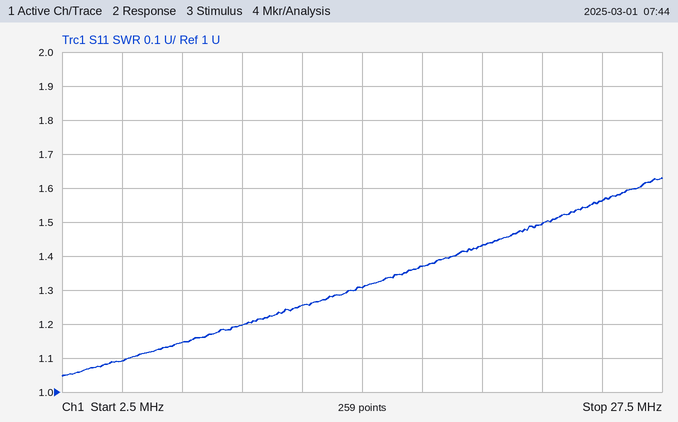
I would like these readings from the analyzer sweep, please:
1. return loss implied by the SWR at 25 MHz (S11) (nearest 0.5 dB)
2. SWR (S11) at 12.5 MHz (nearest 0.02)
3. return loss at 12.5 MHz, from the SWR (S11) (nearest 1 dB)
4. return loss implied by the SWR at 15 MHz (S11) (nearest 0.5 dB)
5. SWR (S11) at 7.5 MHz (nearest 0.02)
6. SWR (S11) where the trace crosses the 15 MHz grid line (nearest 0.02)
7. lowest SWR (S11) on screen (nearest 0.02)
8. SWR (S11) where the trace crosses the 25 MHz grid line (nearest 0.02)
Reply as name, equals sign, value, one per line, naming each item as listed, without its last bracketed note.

return loss implied by the SWR at 25 MHz (S11) = 13.0 dB
SWR (S11) at 12.5 MHz = 1.26
return loss at 12.5 MHz, from the SWR (S11) = 19 dB
return loss implied by the SWR at 15 MHz (S11) = 17.5 dB
SWR (S11) at 7.5 MHz = 1.14
SWR (S11) where the trace crosses the 15 MHz grid line = 1.30
lowest SWR (S11) on screen = 1.04
SWR (S11) where the trace crosses the 25 MHz grid line = 1.56
